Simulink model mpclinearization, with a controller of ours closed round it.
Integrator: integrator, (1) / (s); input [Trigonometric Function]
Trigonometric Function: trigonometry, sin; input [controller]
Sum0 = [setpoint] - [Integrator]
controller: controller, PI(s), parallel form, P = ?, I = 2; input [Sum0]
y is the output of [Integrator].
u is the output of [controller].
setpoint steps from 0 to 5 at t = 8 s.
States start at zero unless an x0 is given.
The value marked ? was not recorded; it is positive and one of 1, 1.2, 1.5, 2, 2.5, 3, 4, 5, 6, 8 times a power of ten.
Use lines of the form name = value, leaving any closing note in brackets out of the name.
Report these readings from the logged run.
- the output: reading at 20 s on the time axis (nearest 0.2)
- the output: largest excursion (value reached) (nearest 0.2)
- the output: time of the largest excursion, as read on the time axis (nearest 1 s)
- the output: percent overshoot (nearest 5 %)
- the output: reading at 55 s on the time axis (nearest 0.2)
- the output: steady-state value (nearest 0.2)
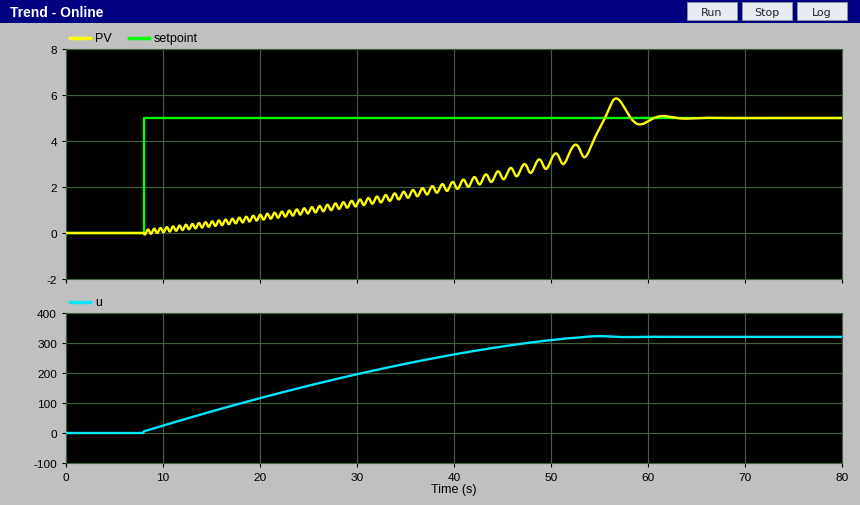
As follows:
the output: reading at 20 s on the time axis = 0.8
the output: largest excursion (value reached) = 5.8
the output: time of the largest excursion, as read on the time axis = 57 s
the output: percent overshoot = 15 %
the output: reading at 55 s on the time axis = 4.6
the output: steady-state value = 5.0
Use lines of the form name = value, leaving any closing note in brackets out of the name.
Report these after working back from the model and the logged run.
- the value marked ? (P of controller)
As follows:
the value marked ? = 1
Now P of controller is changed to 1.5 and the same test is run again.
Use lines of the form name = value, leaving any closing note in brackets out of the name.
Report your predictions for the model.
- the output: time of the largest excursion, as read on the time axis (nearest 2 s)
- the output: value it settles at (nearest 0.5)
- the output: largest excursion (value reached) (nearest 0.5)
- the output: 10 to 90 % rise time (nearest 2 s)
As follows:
the output: time of the largest excursion, as read on the time axis = 42 s
the output: value it settles at = 5.0
the output: largest excursion (value reached) = 5.5
the output: 10 to 90 % rise time = 28 s
